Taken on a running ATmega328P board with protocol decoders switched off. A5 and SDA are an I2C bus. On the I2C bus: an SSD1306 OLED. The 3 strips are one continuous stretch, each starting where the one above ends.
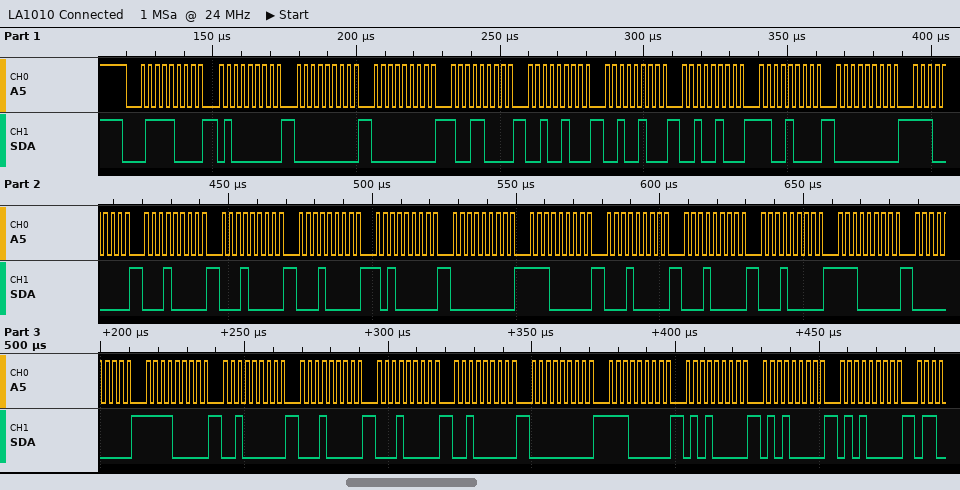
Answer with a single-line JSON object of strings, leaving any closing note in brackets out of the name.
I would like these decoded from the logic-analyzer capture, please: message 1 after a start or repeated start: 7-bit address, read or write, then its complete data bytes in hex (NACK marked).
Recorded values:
{"message 1 after a start or repeated start: 7-bit address, read or write, then its complete data bytes in hex": "0x3C write: 40 00 00 98 24 24 24 C8 00 E0 10 10 10 A0 00 E0 10 10 10 E0 00 F0 20 10 10 20 00 E0 50 50 50"}
